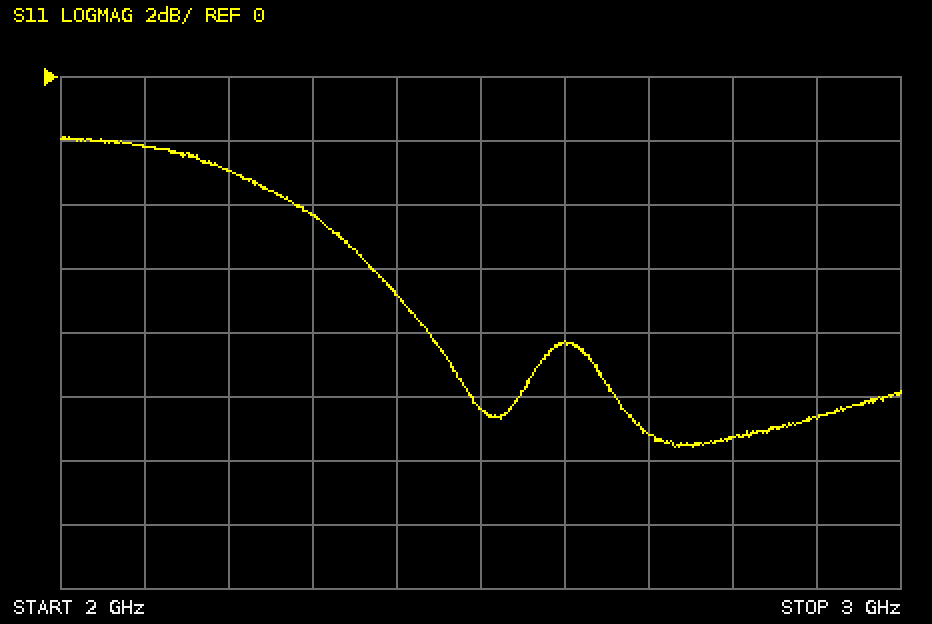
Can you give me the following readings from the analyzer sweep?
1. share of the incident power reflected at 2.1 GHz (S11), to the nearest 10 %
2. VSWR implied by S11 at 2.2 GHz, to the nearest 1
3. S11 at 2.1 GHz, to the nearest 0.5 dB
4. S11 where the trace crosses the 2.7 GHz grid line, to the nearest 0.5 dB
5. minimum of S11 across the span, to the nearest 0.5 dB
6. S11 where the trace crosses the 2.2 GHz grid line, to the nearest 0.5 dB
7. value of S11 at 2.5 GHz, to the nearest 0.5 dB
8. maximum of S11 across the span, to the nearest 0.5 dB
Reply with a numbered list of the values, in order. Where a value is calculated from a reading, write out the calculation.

1. 10^(-2/10) ≈ 63.1 %, so 60 % to the nearest 10 %
2. |Γ| = 10^(-3/20) = 0.7079; VSWR = (1 + 0.7079)/(1 − 0.7079) ≈ 6
3. -2.0 dB
4. -11.0 dB
5. -11.5 dB
6. -3.0 dB
7. -10.5 dB
8. -2.0 dB
